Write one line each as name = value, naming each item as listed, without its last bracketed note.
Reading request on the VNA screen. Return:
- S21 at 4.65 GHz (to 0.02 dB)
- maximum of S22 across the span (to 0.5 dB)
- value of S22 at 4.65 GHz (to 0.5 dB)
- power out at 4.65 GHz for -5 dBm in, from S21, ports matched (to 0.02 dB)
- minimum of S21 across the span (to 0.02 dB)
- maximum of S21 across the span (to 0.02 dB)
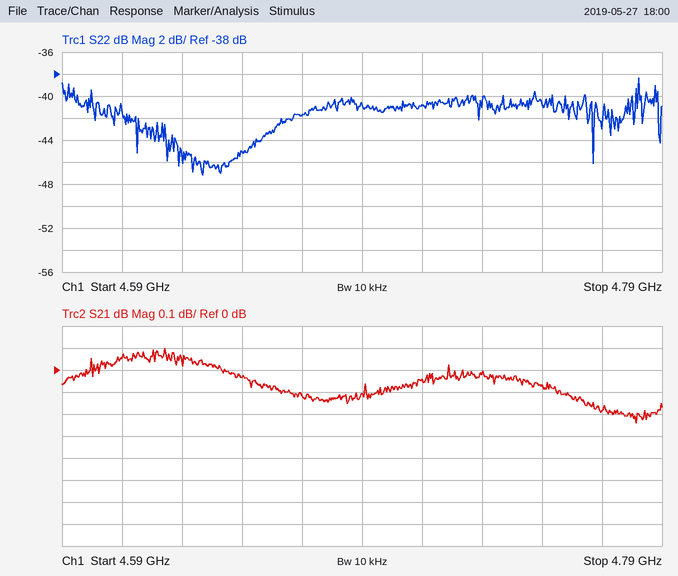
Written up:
S21 at 4.65 GHz = -0.04 dB
maximum of S22 across the span = -38.5 dB
value of S22 at 4.65 GHz = -45.0 dB
power out at 4.65 GHz for -5 dBm in, from S21, ports matched = -5.04 dBm
minimum of S21 across the span = -0.24 dB
maximum of S21 across the span = 0.10 dB
